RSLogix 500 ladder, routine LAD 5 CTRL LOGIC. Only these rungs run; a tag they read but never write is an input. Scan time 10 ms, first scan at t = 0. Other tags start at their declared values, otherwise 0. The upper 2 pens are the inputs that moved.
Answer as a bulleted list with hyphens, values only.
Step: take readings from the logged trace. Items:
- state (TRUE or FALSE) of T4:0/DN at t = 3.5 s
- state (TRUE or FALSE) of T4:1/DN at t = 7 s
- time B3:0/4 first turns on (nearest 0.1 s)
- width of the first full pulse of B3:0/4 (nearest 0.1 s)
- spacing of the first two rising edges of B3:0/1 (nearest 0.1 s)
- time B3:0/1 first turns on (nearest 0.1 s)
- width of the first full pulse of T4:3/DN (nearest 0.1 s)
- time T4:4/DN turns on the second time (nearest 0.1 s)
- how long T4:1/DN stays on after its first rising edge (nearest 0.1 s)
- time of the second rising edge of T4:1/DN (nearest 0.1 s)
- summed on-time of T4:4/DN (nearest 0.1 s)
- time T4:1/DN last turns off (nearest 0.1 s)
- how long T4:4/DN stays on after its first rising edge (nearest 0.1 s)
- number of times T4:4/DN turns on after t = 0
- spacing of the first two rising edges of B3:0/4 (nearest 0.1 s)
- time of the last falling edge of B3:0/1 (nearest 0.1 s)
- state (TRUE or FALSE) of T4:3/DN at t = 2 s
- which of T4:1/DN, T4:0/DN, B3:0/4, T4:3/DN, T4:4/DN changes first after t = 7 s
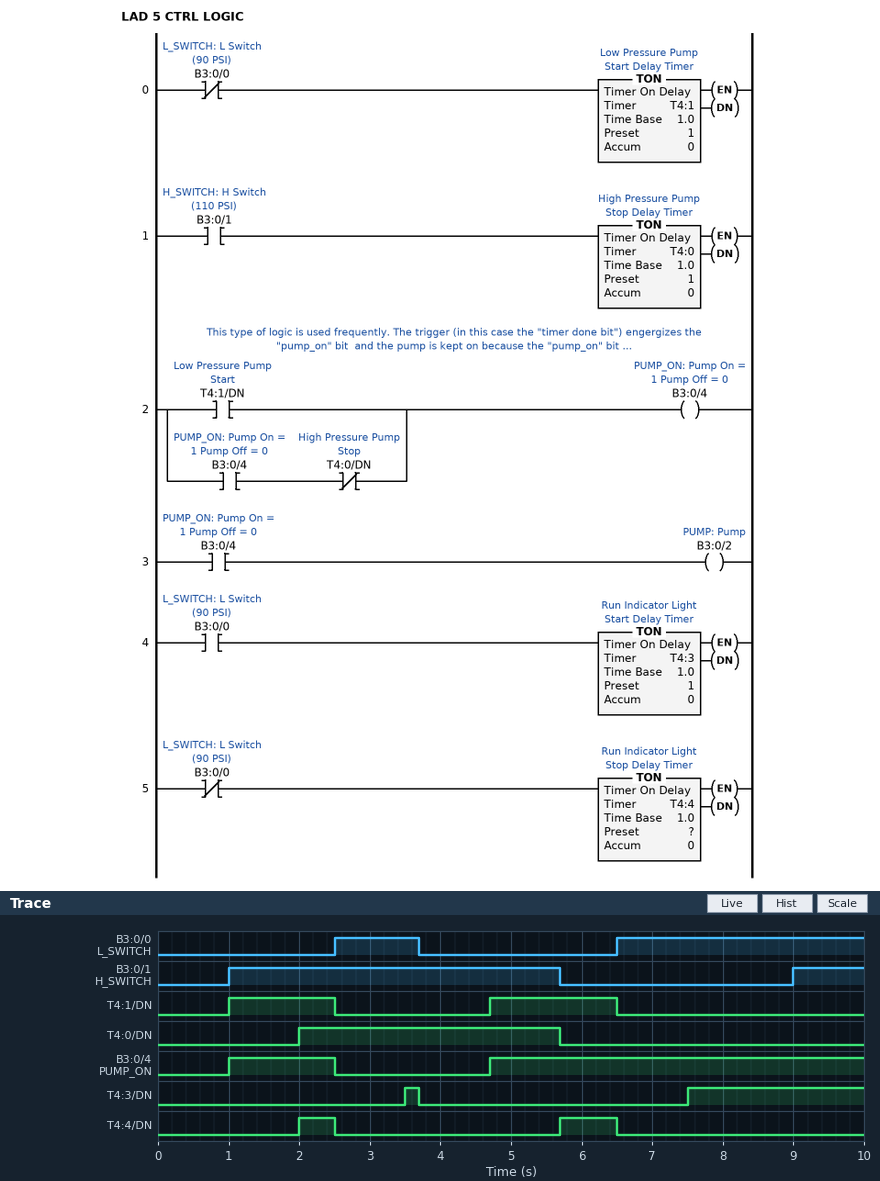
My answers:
- TRUE
- FALSE
- 1.0 s
- 1.5 s
- 8.0 s
- 1.0 s
- 0.2 s
- 5.7 s
- 1.5 s
- 4.7 s
- 1.3 s
- 6.5 s
- 0.5 s
- 2
- 3.7 s
- 5.7 s
- FALSE
- T4:3/DN
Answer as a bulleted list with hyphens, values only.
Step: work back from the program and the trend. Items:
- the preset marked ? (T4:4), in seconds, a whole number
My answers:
- 2 s
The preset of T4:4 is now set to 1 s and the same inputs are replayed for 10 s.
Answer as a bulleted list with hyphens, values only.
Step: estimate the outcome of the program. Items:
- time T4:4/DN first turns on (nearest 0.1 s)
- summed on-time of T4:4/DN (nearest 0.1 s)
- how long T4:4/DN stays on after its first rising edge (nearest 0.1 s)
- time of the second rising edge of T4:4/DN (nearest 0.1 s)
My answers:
- 1.0 s
- 3.3 s
- 1.5 s
- 4.7 s
